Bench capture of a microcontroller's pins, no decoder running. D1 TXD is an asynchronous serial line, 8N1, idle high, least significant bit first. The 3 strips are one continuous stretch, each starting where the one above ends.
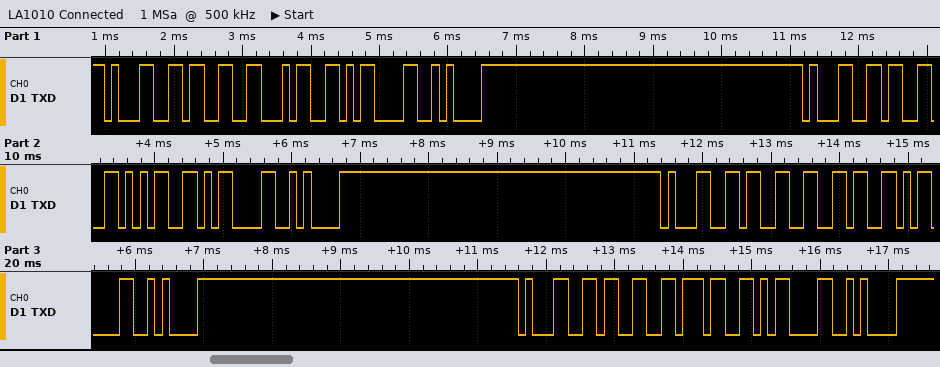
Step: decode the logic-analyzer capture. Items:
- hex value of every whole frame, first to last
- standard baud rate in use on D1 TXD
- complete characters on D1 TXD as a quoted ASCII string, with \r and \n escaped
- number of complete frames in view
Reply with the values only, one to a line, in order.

0x31 0x33 0x34 0x0D 0x0A 0x31 0x33 0x35 0x0D 0x0A 0x31 0x33 0x36 0x0D 0x0A 0x31 0x33 0x37 0x0D 0x0A
9600 baud
"134\r\n135\r\n136\r\n137\r\n"
20
